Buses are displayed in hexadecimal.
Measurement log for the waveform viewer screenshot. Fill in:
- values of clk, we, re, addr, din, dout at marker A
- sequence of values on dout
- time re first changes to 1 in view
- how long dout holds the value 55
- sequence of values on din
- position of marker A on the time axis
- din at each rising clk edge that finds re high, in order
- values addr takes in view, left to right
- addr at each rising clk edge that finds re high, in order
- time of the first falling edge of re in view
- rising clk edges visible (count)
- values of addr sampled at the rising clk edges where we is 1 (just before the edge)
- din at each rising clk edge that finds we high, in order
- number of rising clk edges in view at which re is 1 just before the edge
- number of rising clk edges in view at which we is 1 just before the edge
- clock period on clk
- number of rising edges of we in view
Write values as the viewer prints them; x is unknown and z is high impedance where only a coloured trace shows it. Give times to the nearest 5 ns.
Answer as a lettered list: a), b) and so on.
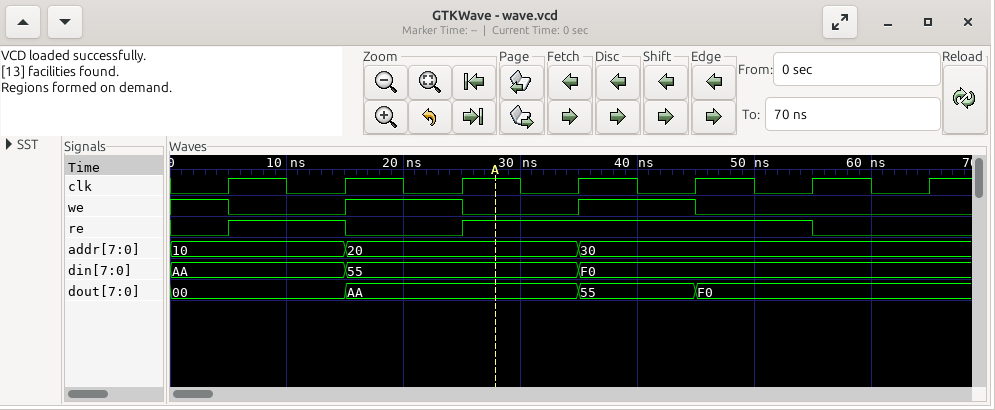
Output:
a) clk=1, we=0, re=1, addr=20, din=55, dout=AA
b) 00, AA, 55, F0
c) 5 ns
d) 10 ns
e) AA, 55, F0
f) 30 ns
g) AA, 55, F0, F0
h) 10, 20, 30
i) 10, 20, 30, 30
j) 15 ns
k) 7
l) 10, 20, 30
m) AA, 55, F0
n) 4
o) 3
p) 10 ns
q) 2
